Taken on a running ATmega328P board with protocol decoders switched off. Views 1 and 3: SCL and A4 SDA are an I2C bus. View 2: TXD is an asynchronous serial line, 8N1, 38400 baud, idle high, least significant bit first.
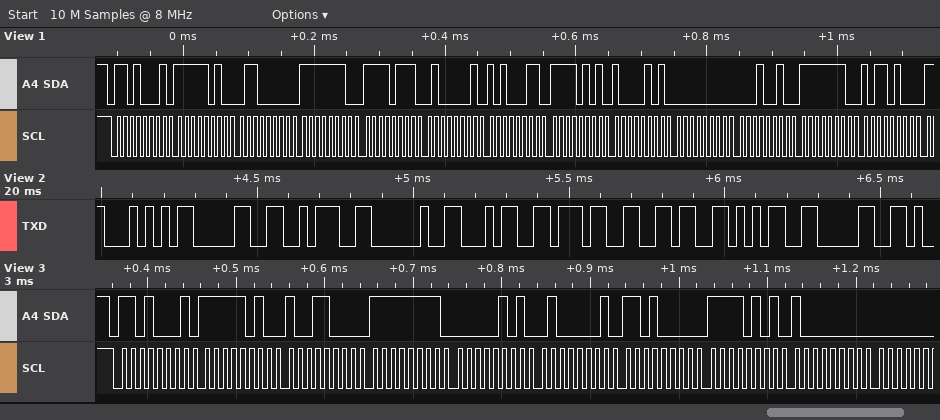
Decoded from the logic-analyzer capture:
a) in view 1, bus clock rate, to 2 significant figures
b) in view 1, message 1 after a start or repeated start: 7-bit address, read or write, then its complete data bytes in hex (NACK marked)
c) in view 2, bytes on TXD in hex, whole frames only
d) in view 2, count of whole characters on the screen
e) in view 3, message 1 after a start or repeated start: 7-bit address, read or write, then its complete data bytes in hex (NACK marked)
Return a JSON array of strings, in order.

["100 kHz", "0x68 read: FA 60 FE F7 41 A3 F5 85 00 12 FE B4", "54 30 3A 20 34 37 36 35 30", "9", "0x68 read: FA 98 FF 05 41 D0 F5 80"]
